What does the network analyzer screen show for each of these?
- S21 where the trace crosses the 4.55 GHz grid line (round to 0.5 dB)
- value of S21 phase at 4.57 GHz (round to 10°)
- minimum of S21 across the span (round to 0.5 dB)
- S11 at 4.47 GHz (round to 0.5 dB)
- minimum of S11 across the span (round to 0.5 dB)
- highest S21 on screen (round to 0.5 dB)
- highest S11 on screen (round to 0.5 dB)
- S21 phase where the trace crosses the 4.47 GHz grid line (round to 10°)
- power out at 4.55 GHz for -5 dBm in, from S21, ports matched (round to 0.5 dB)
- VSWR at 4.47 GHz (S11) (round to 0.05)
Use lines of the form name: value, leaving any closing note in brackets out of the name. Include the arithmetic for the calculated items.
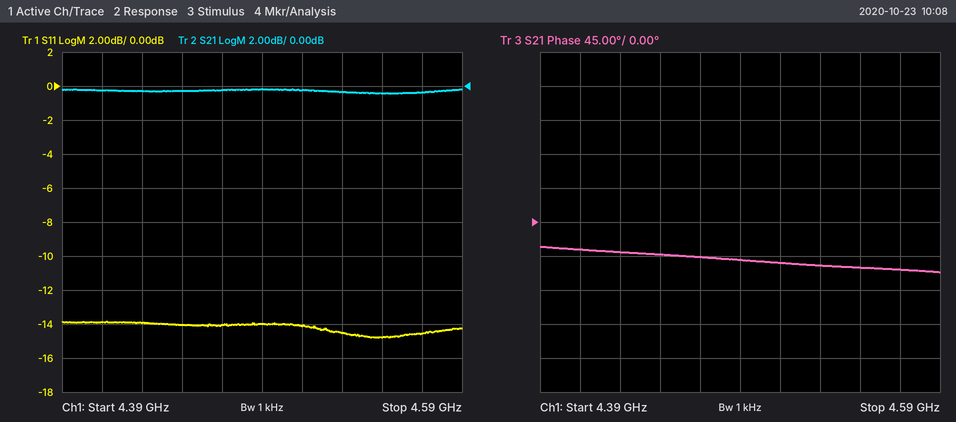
S21 where the trace crosses the 4.55 GHz grid line: -0.5 dB
value of S21 phase at 4.57 GHz: -60°
minimum of S21 across the span: -0.5 dB
S11 at 4.47 GHz: -14.0 dB
minimum of S11 across the span: -15.0 dB
highest S21 on screen: 0.0 dB
highest S11 on screen: -14.0 dB
S21 phase where the trace crosses the 4.47 GHz grid line: -50°
power out at 4.55 GHz for -5 dBm in, from S21, ports matched: -5 dBm + (-0.5 dB) = -5.5 dBm
VSWR at 4.47 GHz (S11): |Γ| = 10^(-14/20) = 0.1995; VSWR = (1 + 0.1995)/(1 − 0.1995) ≈ 1.50
